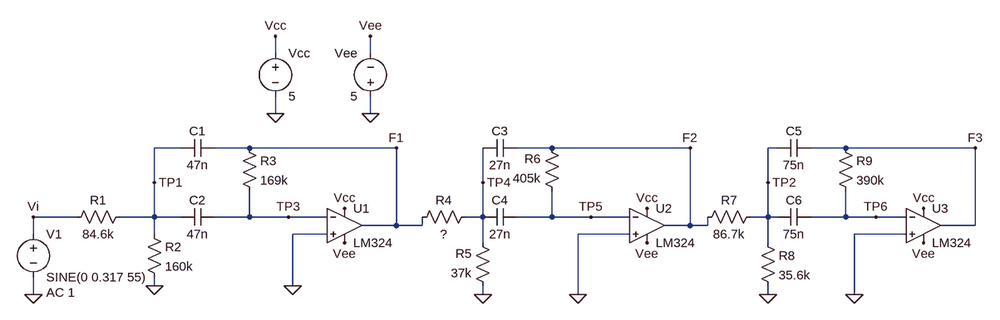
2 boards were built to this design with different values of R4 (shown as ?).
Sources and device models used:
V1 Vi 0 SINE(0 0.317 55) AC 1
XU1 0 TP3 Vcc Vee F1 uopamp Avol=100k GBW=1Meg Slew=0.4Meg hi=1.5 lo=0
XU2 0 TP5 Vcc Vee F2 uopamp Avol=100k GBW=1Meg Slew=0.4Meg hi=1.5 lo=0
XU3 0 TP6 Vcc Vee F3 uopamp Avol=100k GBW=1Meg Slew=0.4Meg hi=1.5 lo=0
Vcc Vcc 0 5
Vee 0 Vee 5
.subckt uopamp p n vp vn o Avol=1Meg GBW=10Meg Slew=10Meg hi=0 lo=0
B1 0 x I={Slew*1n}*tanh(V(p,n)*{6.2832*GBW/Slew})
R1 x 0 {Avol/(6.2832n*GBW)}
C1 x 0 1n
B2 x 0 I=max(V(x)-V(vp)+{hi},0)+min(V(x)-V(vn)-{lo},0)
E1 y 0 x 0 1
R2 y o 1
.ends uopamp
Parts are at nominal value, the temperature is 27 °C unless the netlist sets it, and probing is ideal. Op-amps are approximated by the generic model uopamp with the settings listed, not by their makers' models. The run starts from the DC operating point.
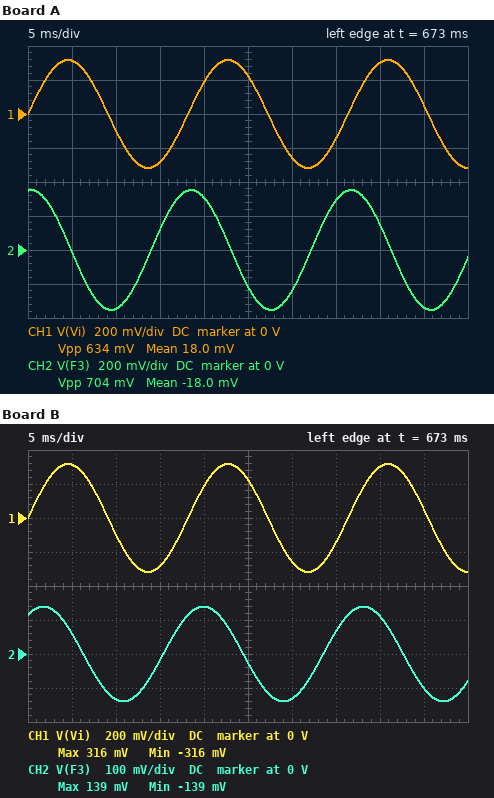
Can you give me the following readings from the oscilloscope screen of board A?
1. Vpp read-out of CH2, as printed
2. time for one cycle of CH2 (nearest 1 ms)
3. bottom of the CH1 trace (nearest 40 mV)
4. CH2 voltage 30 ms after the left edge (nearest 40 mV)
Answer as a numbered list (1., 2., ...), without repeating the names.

1. 704 mV
2. 18 ms
3. -320 mV
4. -240 mV
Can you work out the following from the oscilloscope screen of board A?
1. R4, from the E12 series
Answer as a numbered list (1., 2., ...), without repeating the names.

1. 68 kΩ
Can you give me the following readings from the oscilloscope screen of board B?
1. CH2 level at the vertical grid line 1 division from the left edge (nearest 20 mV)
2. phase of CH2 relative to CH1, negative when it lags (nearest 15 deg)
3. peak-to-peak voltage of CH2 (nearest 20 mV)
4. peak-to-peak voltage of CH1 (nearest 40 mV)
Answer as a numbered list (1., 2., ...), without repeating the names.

1. 60 mV
2. 60 deg
3. 280 mV
4. 640 mV
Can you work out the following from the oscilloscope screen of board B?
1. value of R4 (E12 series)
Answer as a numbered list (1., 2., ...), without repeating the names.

1. 180 kΩ
